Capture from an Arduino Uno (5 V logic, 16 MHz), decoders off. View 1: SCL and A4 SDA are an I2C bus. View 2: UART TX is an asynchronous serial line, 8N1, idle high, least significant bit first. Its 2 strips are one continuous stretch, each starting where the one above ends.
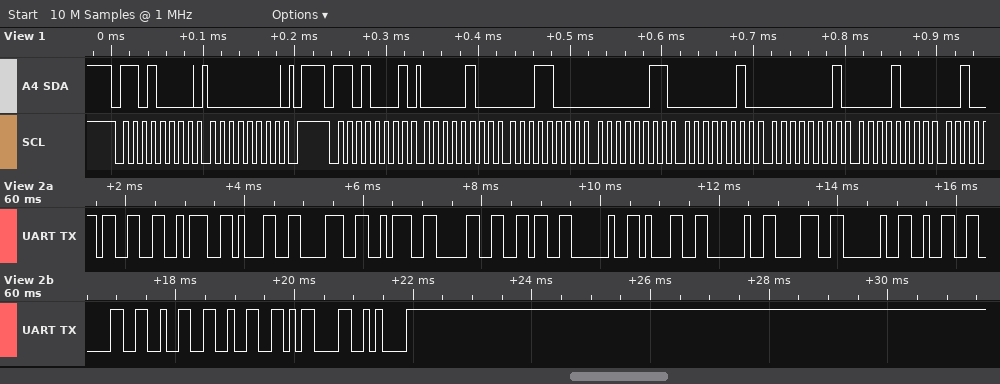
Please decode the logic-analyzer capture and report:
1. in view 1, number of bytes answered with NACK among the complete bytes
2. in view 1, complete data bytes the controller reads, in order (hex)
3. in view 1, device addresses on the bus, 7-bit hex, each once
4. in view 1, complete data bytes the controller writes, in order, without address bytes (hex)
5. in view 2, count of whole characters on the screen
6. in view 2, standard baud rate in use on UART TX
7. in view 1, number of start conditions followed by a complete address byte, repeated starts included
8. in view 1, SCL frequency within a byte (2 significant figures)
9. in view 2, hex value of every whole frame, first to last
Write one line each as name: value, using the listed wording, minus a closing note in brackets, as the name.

in view 1, number of bytes answered with NACK among the complete bytes: 0
in view 1, complete data bytes the controller reads, in order: 04 18 03 02 01 08
in view 1, device addresses on the bus, 7-bit hex, each once: 0x68
in view 1, complete data bytes the controller writes, in order, without address bytes: 00
in view 2, count of whole characters on the screen: 18
in view 2, standard baud rate in use on UART TX: 9600 baud
in view 1, number of start conditions followed by a complete address byte, repeated starts included: 2
in view 1, SCL frequency within a byte: 100 kHz
in view 2, hex value of every whole frame, first to last: 33 3A 31 38 3A 30 36 20 31 20 38 20 32 30 32 32 0D 0A
